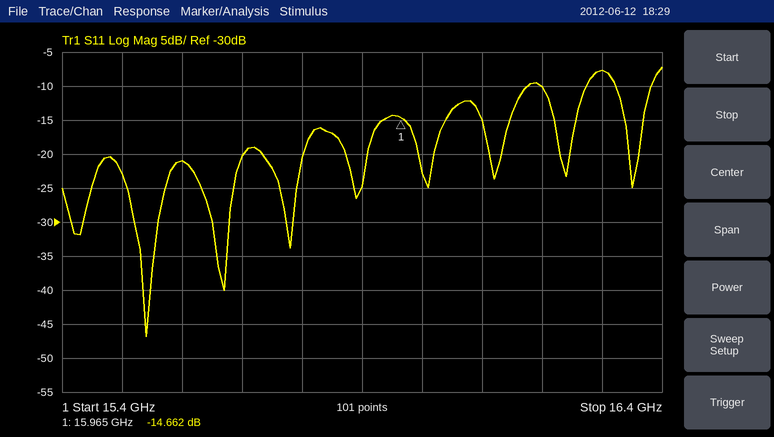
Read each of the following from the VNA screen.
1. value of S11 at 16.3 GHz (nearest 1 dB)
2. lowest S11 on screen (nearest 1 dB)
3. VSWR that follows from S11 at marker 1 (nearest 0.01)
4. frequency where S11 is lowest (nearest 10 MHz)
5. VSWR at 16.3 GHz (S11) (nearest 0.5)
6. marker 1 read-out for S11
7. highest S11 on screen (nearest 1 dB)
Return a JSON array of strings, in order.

["-8 dB", "-47 dB", "1.45", "15.54 GHz", "2.5", "-14.662 dB", "-7 dB"]
